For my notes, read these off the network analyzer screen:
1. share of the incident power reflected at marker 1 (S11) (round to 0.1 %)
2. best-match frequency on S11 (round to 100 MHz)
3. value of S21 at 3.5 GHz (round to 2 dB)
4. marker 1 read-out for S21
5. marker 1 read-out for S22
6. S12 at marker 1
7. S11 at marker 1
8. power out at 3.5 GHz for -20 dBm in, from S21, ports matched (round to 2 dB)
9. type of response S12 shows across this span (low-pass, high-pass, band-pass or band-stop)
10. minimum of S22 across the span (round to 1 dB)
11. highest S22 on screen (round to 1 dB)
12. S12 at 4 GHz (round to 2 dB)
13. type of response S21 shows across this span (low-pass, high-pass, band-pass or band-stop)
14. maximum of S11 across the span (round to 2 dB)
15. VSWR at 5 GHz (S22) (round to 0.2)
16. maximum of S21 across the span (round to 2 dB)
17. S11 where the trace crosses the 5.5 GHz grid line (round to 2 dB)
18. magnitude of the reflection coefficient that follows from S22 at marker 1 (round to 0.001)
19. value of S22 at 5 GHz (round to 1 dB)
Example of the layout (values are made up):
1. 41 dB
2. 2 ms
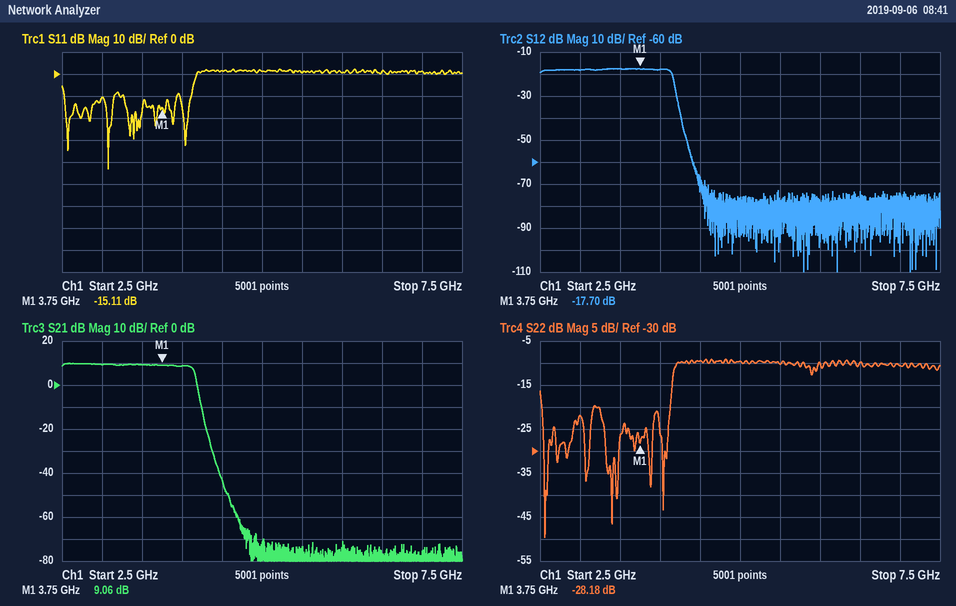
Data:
1. 3.1 %
2. 3.1 GHz
3. 10 dB
4. 9.06 dB
5. -28.18 dB
6. -17.70 dB
7. -15.11 dB
8. -10 dBm
9. low-pass
10. -50 dB
11. -9 dB
12. -18 dB
13. low-pass
14. 2 dB
15. 2.0
16. 10 dB
17. 0 dB
18. 0.039
19. -10 dB
